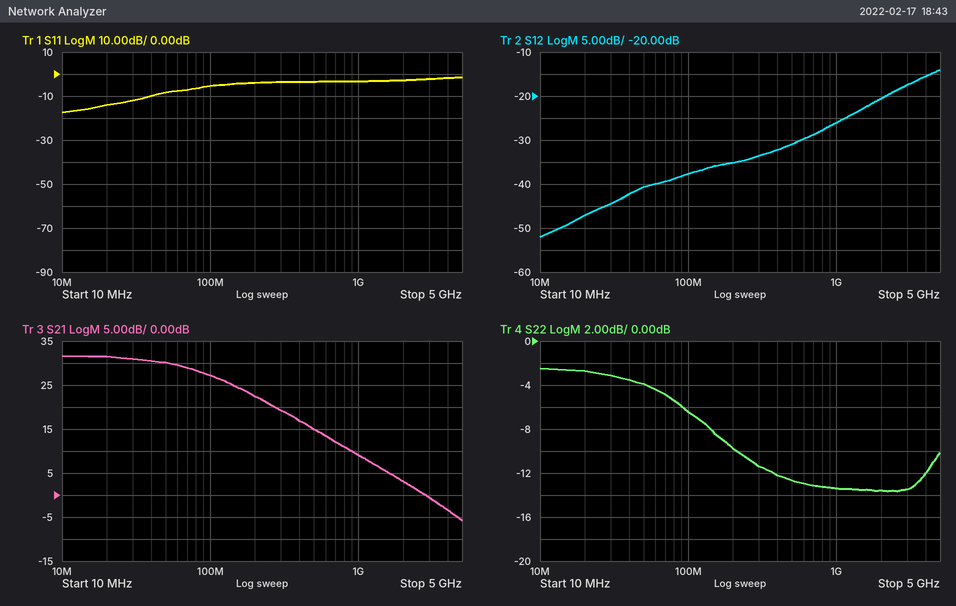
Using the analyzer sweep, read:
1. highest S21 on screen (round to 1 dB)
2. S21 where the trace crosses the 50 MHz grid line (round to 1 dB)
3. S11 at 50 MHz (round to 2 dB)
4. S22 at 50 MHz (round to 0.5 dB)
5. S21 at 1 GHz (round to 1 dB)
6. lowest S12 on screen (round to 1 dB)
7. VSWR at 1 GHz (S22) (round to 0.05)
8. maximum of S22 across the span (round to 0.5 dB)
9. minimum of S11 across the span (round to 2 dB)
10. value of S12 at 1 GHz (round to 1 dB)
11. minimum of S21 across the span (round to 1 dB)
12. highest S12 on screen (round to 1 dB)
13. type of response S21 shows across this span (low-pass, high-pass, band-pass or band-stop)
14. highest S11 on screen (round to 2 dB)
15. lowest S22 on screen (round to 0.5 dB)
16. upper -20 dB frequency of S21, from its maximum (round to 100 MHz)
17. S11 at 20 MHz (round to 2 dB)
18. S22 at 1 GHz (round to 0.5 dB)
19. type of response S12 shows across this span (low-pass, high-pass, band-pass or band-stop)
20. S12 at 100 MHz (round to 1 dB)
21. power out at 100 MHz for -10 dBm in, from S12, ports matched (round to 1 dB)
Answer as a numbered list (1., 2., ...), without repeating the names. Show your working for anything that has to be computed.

1. 32 dB
2. 30 dB
3. -8 dB
4. -4.0 dB
5. 9 dB
6. -52 dB
7. |Γ| = 10^(-13.5/20) = 0.2113; VSWR = (1 + 0.2113)/(1 − 0.2113) ≈ 1.54, so 1.55 to the nearest 0.05
8. -2.5 dB
9. -18 dB
10. -26 dB
11. -6 dB
12. -14 dB
13. low-pass
14. -2 dB
15. -13.5 dB
16. 700 MHz
17. -14 dB
18. -13.5 dB
19. high-pass
20. -38 dB
21. -10 dBm + (-38 dB) = -48 dBm
